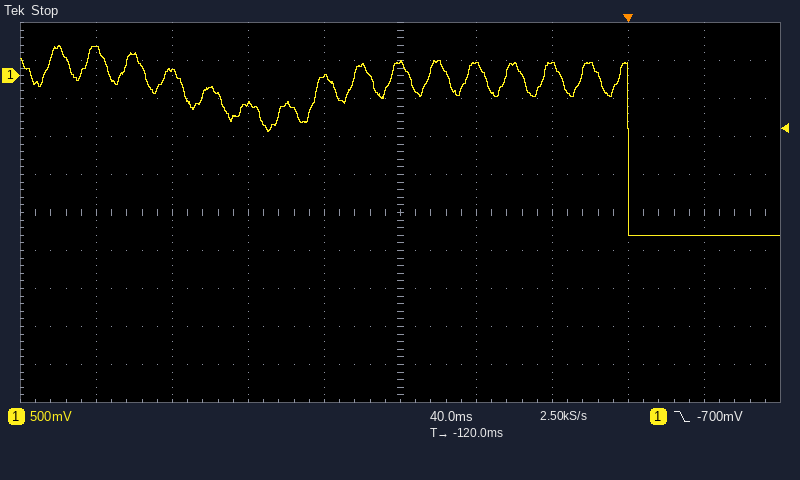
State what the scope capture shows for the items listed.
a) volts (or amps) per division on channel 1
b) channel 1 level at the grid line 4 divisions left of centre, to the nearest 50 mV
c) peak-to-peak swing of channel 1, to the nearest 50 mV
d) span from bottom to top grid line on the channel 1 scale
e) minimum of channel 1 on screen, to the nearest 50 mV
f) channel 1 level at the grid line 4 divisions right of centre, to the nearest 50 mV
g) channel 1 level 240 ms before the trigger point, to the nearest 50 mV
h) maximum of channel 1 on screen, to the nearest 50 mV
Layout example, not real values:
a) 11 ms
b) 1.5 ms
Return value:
a) 500 mV
b) 350 mV
c) 2.50 V
d) 5 V
e) -2.10 V
f) -2.10 V
g) 50 mV
h) 400 mV
